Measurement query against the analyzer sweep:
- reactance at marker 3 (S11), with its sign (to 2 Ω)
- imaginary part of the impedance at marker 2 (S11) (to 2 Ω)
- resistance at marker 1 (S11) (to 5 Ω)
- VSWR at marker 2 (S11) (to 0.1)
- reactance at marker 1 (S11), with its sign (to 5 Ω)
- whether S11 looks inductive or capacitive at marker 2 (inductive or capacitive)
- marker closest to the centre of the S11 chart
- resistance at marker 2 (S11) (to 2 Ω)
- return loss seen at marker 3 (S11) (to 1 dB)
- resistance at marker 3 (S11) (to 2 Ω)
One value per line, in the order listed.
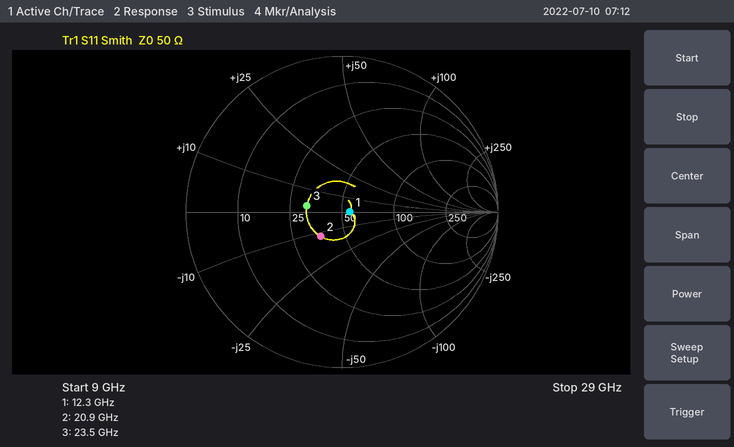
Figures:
+2 Ω
-12 Ω
55 Ω
1.5
0 Ω
capacitive
marker 1
36 Ω
13 dB
32 Ω
